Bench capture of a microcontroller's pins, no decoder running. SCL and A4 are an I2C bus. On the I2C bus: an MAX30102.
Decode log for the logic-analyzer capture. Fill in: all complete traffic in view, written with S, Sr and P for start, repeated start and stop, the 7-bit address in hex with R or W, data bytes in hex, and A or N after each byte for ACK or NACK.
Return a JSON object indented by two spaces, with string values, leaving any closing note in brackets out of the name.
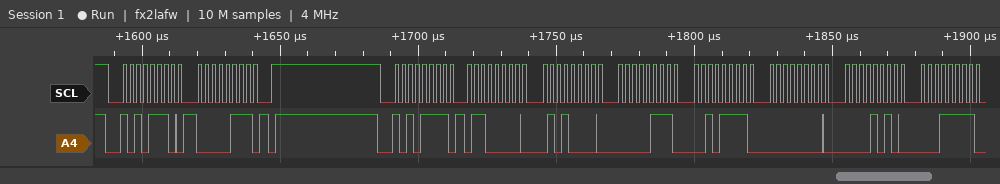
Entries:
{
  "all complete traffic in view, written with S, Sr and P for start, repeated start and stop, the 7-bit address in hex with R or W, data bytes in hex, and A or N after each byte for ACK or NACK": "S 57W A 07 A P S 57R A 60 A 50 A 07 A 2F A 00 A 0A A 1F A"
}
